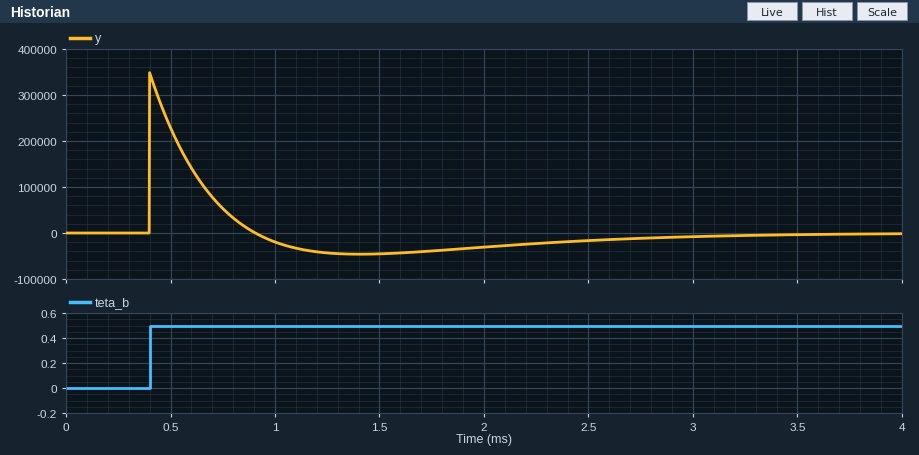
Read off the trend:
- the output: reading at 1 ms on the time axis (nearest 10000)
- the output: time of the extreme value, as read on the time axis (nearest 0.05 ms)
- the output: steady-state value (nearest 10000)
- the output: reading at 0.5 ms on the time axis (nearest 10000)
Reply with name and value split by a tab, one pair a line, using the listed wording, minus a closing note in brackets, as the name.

the output: reading at 1 ms on the time axis	-20000
the output: time of the extreme value, as read on the time axis	0.40 ms
the output: steady-state value	0
the output: reading at 0.5 ms on the time axis	230000
